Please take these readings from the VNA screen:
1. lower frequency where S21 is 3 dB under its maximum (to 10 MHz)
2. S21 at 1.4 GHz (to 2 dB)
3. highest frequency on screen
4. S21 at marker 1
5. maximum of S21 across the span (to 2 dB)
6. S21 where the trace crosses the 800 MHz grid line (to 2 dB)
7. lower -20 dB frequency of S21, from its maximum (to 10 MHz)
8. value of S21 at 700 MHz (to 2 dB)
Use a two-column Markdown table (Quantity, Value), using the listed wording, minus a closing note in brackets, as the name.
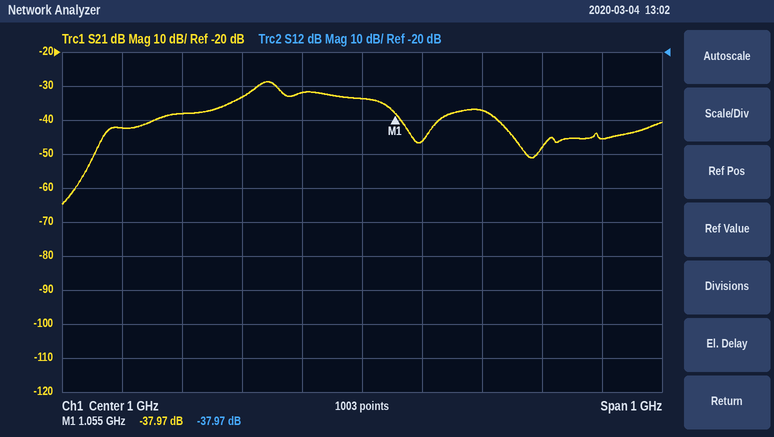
| Quantity | Value |
|---|---|
| lower frequency where S21 is 3 dB under its maximum | 810 MHz |
| S21 at 1.4 GHz | -46 dB |
| highest frequency on screen | 1.5 GHz |
| S21 at marker 1 | -37.97 dB |
| maximum of S21 across the span | -28 dB |
| S21 where the trace crosses the 800 MHz grid line | -34 dB |
| lower -20 dB frequency of S21, from its maximum | 560 MHz |
| value of S21 at 700 MHz | -38 dB |
